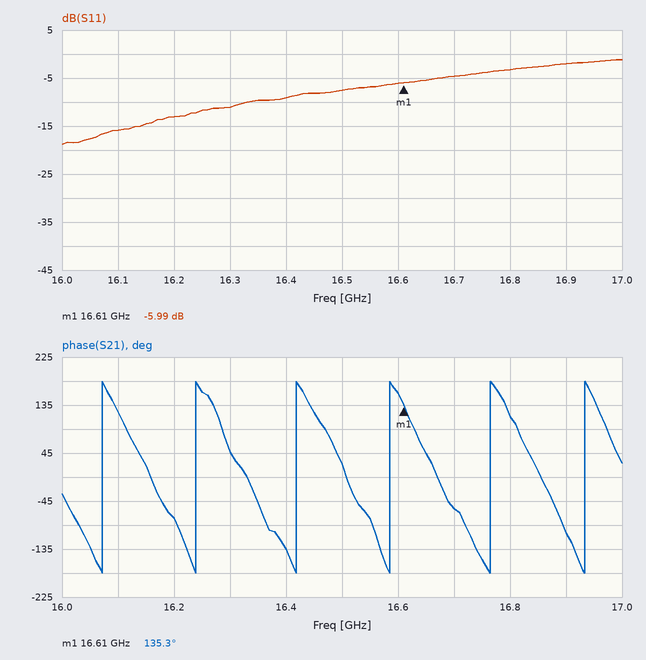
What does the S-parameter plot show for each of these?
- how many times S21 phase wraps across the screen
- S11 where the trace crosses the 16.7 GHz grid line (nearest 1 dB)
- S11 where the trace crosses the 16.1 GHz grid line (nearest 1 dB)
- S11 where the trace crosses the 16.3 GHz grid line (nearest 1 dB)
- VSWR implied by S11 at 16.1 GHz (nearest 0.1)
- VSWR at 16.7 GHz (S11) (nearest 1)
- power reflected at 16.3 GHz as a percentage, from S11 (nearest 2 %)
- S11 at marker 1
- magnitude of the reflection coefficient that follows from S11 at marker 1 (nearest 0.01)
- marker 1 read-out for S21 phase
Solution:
6
-5 dB
-16 dB
-11 dB
1.4
4
8 %
-5.99 dB
0.50
135.3°
